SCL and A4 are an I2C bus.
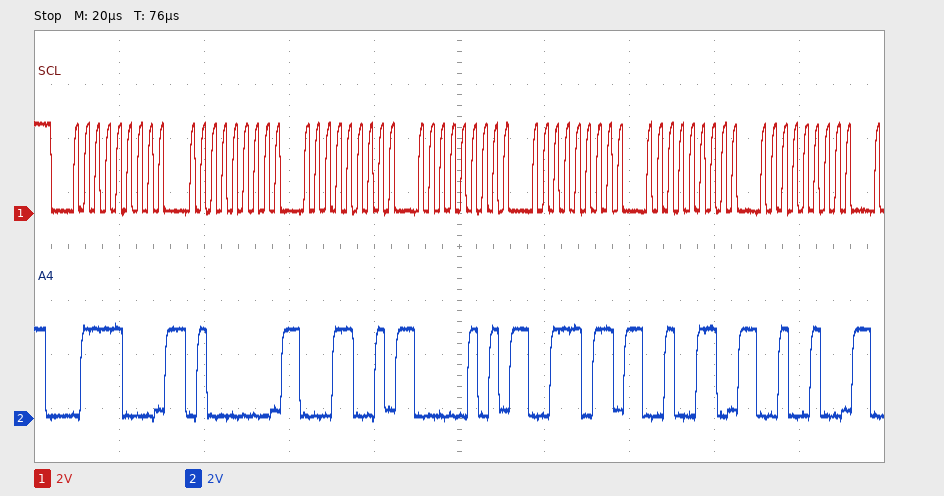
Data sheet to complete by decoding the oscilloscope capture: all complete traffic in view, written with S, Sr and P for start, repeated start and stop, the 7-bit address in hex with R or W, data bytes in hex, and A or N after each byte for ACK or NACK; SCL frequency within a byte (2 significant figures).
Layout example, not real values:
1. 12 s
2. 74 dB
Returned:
1. S 3CW A 40 A 19 A 05 A 3B A 26 A 24 A
2. 400 kHz
